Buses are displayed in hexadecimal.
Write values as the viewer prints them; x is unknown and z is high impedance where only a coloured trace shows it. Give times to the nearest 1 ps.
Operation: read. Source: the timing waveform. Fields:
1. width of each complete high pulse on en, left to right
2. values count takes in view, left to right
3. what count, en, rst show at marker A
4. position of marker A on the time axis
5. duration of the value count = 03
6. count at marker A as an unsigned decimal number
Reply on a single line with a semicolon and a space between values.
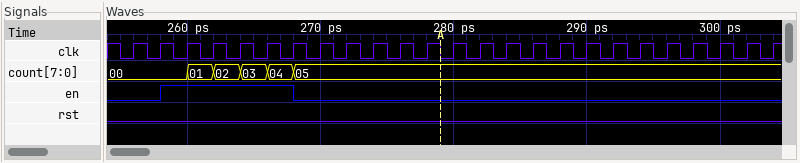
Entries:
10 ps; 00, 01, 02, 03, 04, 05; count=05, en=0, rst=0; 279 ps; 2 ps; 5
